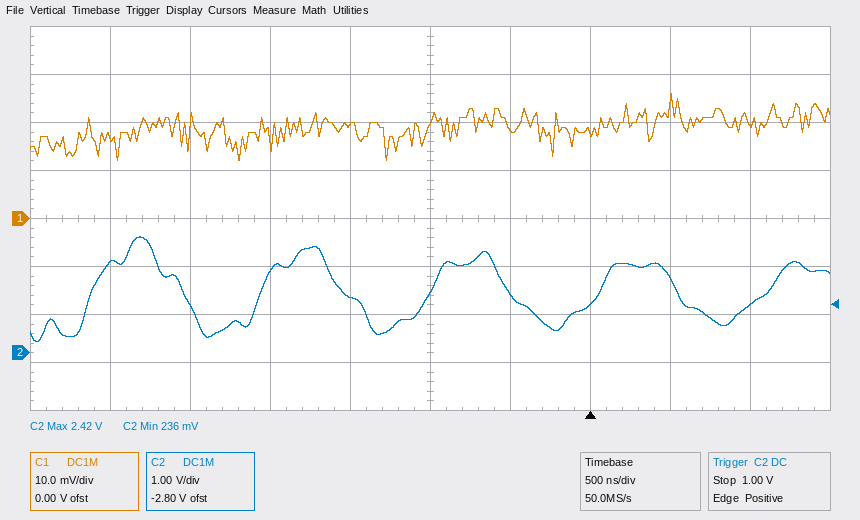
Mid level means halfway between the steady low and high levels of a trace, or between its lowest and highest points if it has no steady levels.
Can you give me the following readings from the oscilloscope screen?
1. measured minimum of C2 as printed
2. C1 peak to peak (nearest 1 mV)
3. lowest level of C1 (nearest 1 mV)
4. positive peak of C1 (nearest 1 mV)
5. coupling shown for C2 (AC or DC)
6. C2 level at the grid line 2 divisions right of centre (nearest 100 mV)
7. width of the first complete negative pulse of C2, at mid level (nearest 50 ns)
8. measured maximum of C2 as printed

236 mV
14 mV
12 mV
26 mV
DC
1.0 V
500 ns
2.42 V
